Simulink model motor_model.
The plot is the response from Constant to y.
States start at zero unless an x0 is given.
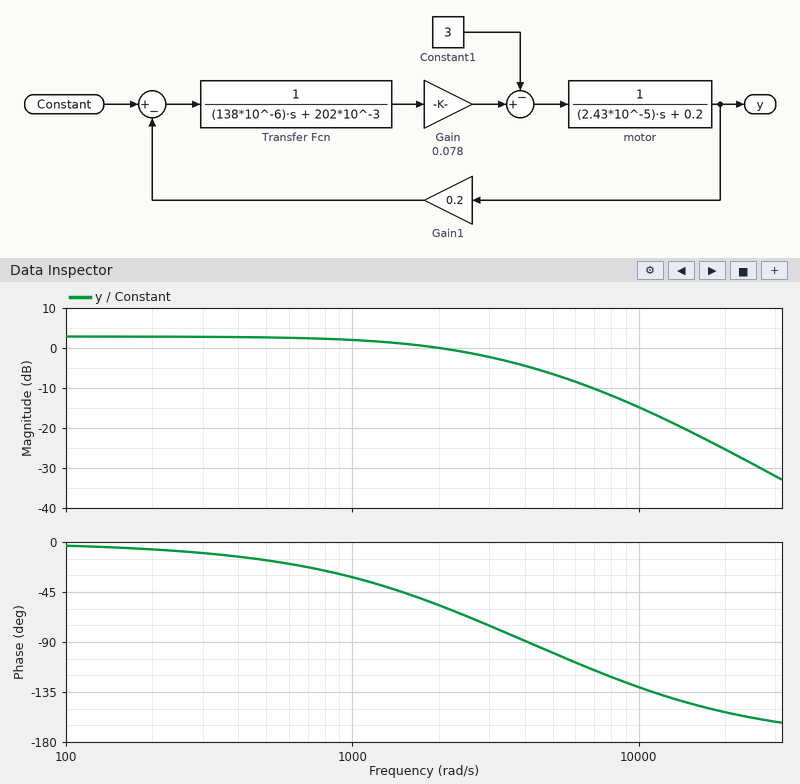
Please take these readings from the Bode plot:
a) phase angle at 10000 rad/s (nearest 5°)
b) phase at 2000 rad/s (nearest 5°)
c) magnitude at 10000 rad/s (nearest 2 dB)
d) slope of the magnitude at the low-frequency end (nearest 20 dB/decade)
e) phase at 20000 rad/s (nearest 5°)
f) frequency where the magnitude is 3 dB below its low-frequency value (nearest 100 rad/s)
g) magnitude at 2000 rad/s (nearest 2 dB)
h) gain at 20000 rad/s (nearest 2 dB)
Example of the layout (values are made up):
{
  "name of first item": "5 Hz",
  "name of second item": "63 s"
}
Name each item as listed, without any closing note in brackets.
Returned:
{
  "phase angle at 10000 rad/s": "-130°",
  "phase at 2000 rad/s": "-55°",
  "magnitude at 10000 rad/s": "-14 dB",
  "slope of the magnitude at the low-frequency end": "0 dB/decade",
  "phase at 20000 rad/s": "-155°",
  "frequency where the magnitude is 3 dB below its low-frequency value": "2100 rad/s",
  "magnitude at 2000 rad/s": "0 dB",
  "gain at 20000 rad/s": "-26 dB"
}
